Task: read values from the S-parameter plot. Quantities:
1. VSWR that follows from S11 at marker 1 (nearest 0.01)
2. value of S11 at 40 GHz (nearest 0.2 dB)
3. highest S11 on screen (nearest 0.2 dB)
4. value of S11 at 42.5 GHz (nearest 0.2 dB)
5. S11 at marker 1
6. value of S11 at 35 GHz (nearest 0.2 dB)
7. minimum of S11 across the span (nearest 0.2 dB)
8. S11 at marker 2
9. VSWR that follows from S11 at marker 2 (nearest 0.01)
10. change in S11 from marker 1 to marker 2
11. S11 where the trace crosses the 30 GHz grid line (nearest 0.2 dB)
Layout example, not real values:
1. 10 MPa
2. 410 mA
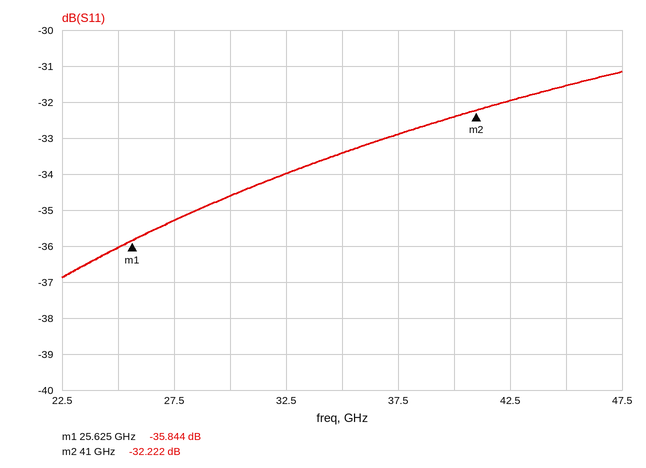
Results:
1. 1.03
2. -32.4 dB
3. -31.2 dB
4. -32.0 dB
5. -35.844 dB
6. -33.4 dB
7. -36.8 dB
8. -32.222 dB
9. 1.05
10. 3.622 dB
11. -34.6 dB
